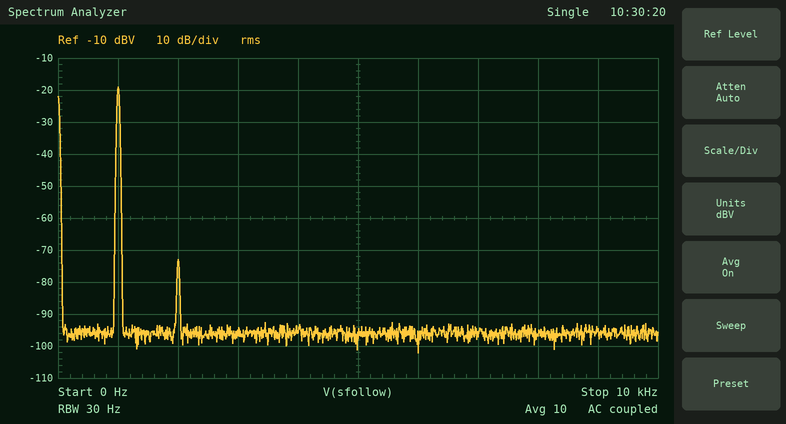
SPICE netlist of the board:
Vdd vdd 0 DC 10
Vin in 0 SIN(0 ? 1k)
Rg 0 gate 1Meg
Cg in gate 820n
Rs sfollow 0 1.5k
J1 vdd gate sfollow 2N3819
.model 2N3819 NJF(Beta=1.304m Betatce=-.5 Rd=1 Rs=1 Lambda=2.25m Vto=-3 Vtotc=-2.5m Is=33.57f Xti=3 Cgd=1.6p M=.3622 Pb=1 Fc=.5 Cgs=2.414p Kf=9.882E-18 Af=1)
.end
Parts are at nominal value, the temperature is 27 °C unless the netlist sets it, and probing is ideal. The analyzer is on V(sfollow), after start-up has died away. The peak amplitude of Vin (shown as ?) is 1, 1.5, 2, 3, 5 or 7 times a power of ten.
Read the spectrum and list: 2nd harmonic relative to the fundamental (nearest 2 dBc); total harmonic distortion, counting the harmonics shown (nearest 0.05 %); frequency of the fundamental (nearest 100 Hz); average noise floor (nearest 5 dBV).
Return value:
-54 dBc
0.20 %
1.0 kHz
-95 dBV
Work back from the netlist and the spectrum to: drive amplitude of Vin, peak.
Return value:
200 mV
